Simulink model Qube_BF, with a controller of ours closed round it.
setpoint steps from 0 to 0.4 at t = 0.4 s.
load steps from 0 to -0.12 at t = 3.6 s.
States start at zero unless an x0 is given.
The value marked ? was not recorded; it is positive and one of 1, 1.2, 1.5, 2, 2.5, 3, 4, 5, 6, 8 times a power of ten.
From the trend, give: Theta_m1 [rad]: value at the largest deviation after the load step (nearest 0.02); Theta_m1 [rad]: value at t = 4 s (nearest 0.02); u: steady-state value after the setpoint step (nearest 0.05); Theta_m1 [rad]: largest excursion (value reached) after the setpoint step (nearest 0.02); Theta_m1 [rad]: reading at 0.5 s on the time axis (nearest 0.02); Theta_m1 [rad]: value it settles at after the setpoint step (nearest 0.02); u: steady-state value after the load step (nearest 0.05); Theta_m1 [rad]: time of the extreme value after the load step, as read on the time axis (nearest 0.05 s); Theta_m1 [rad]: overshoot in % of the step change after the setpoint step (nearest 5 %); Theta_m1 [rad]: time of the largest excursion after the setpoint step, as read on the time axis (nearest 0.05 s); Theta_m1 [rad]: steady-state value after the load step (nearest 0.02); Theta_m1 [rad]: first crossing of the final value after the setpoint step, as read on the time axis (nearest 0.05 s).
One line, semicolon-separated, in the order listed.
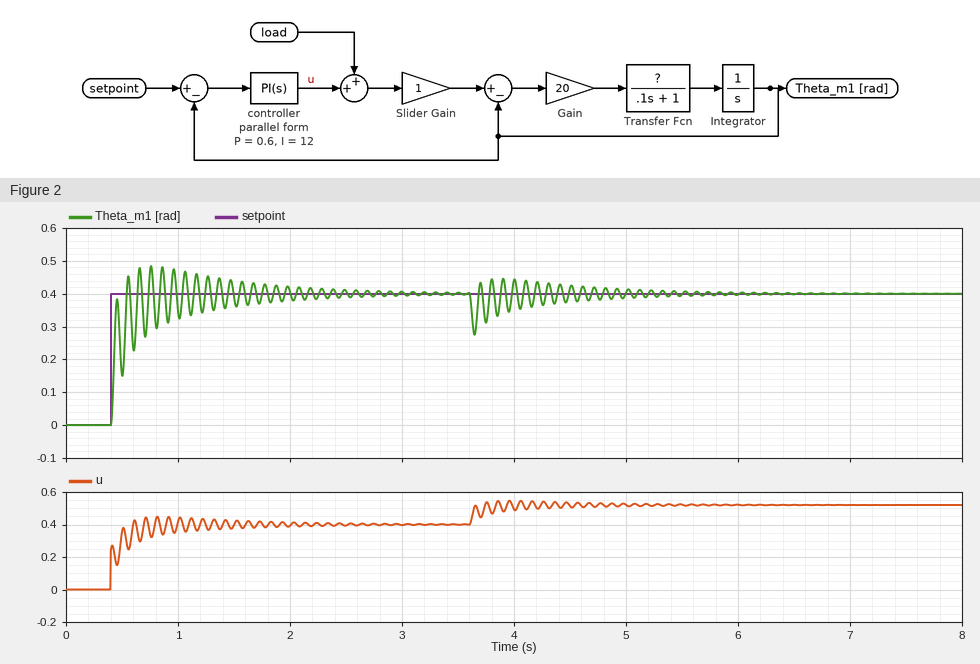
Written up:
0.28; 0.44; 0.40; 0.48; 0.16; 0.40; 0.50; 3.65 s; 20 %; 0.75 s; 0.40; 0.55 s
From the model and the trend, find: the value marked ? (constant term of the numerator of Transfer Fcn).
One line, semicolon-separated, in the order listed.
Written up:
12
